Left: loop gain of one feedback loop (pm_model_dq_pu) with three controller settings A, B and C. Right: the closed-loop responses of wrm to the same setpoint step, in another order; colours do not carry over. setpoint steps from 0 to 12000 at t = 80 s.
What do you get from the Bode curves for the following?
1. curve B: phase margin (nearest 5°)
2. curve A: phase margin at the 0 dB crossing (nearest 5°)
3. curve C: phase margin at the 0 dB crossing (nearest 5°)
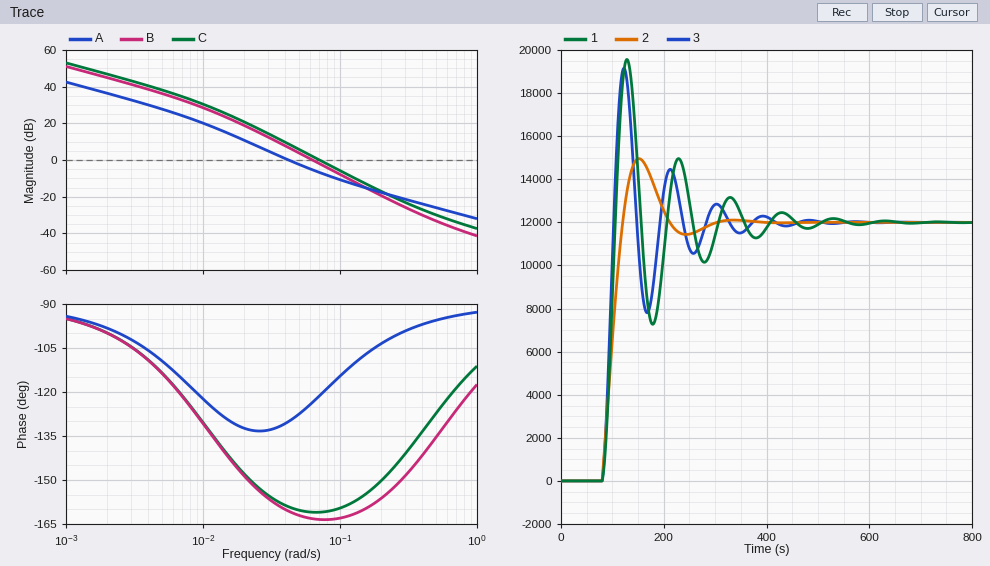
15°
50°
20°
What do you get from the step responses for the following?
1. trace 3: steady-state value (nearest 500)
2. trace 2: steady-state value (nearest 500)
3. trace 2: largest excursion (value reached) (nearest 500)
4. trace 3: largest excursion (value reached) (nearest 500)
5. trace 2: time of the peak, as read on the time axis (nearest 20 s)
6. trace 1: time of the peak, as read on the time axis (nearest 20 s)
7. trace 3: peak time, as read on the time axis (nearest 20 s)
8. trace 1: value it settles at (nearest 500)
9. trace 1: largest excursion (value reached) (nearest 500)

12000
12000
15000
19000
160 s
120 s
120 s
12000
19500
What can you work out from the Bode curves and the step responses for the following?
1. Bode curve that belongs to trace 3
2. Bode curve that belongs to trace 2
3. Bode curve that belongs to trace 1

C
A
B
